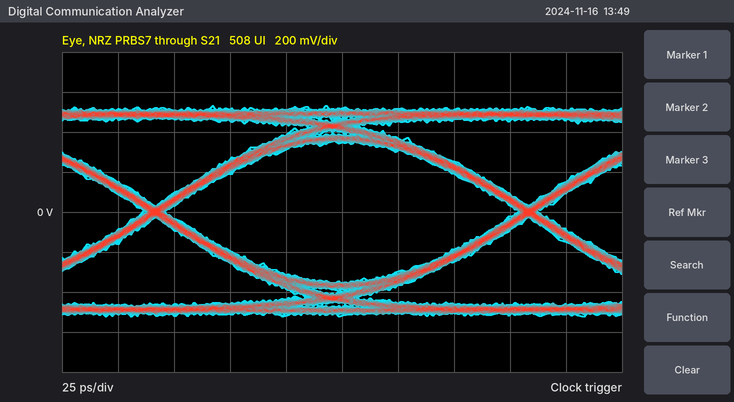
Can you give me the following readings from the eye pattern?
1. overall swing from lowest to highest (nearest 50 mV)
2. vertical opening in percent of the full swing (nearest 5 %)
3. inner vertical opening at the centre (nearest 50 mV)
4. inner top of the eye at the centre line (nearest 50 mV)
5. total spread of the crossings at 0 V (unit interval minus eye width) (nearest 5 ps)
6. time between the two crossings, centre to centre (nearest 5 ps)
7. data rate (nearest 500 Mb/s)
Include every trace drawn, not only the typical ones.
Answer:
1.05 V
65 %
700 mV
350 mV
10 ps
165 ps
6.0 Gb/s
